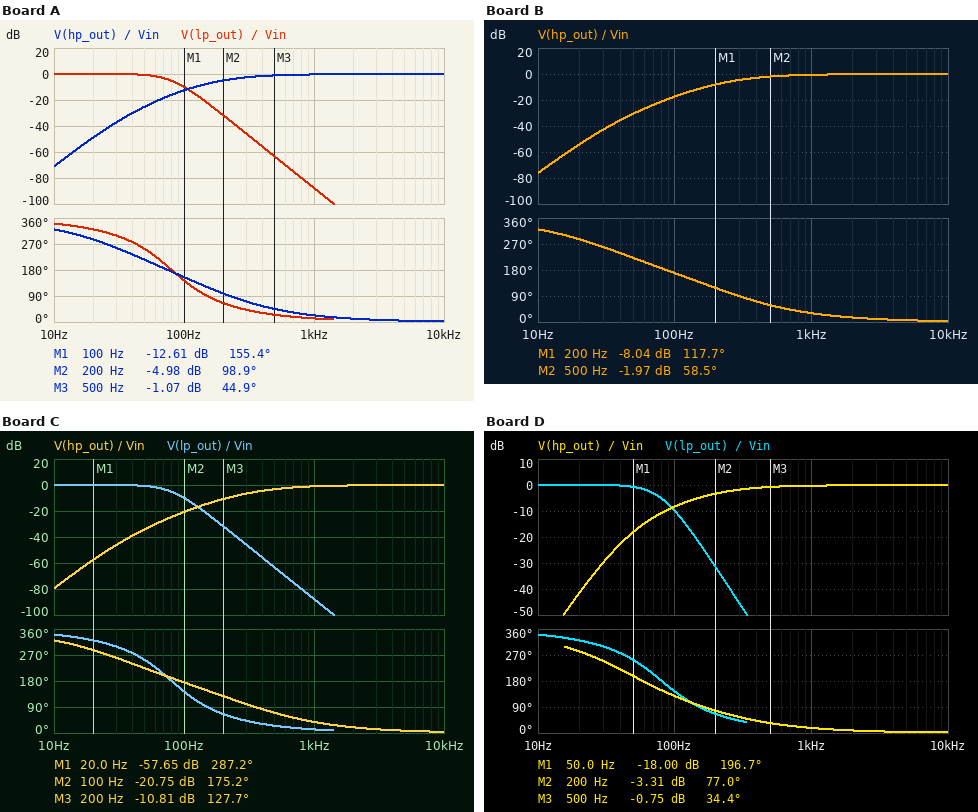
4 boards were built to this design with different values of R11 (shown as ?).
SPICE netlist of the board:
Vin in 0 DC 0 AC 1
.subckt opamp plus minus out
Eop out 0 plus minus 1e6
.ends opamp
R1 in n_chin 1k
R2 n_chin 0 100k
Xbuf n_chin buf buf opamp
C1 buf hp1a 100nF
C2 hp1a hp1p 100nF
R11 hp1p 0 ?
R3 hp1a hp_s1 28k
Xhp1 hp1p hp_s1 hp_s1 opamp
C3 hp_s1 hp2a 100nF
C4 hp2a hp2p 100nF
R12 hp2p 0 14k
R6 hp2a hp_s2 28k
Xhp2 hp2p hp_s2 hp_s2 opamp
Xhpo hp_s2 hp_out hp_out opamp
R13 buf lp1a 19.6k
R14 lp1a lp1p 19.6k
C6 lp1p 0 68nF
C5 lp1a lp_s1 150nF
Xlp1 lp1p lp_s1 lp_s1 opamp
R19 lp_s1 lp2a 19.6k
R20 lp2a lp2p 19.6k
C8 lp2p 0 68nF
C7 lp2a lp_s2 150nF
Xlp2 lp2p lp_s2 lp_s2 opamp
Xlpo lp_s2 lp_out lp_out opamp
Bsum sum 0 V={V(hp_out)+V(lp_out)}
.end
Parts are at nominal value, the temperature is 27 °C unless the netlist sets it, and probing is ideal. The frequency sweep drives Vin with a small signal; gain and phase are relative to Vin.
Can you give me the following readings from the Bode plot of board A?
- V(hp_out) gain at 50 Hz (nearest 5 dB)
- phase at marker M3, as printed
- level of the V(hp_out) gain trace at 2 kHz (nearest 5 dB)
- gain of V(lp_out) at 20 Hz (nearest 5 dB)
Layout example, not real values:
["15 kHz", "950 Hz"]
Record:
["-25 dB", "44.9 deg", "0 dB", "0 dB"]
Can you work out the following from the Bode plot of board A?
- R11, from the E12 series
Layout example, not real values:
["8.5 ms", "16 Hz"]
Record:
["18 kΩ"]
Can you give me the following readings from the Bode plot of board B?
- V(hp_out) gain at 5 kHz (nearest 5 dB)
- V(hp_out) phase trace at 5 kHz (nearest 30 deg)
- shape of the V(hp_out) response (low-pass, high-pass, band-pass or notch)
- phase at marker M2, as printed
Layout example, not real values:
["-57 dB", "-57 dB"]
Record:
["0 dB", "0 deg", "high-pass", "58.5 deg"]
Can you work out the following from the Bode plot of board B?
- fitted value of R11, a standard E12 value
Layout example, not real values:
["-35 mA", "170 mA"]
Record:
["10 kΩ"]
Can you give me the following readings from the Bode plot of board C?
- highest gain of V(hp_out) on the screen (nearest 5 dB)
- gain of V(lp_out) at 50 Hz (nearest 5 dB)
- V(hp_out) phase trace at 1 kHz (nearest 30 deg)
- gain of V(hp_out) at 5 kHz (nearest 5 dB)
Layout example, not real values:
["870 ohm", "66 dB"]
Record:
["0 dB", "0 dB", "30 deg", "0 dB"]
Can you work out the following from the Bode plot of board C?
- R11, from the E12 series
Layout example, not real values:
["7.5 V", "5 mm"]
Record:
["6.8 kΩ"]
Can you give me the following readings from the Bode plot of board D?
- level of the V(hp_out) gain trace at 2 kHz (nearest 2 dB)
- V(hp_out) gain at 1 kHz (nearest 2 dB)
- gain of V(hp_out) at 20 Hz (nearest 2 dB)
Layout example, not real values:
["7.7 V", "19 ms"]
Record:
["0 dB", "0 dB", "-42 dB"]
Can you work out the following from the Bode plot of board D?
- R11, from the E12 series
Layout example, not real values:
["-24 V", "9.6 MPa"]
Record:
["39 kΩ"]
